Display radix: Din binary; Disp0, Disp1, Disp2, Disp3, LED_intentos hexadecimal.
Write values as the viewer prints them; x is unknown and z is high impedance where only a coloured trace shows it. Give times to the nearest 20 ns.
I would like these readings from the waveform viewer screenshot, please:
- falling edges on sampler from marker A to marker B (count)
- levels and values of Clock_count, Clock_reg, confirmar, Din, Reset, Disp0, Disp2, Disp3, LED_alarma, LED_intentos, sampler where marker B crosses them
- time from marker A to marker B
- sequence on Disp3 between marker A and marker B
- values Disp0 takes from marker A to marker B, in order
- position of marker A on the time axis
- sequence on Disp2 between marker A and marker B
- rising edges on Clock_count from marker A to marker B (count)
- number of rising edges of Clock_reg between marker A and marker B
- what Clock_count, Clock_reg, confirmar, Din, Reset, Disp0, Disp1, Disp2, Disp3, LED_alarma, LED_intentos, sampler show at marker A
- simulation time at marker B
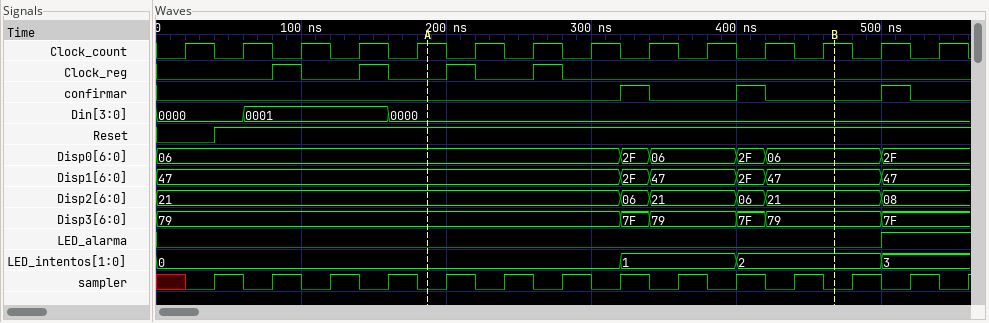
7
Clock_count=1, Clock_reg=0, confirmar=0, Din=0000, Reset=1, Disp0=06, Disp2=21, Disp3=79, LED_alarma=0, LED_intentos=2, sampler=0
280 ns
79, 7F, 79, 7F, 79
06, 2F, 06, 2F, 06
180 ns
21, 06, 21, 06, 21
7
2
Clock_count=1, Clock_reg=0, confirmar=0, Din=0000, Reset=1, Disp0=06, Disp1=47, Disp2=21, Disp3=79, LED_alarma=0, LED_intentos=0, sampler=0
460 ns
